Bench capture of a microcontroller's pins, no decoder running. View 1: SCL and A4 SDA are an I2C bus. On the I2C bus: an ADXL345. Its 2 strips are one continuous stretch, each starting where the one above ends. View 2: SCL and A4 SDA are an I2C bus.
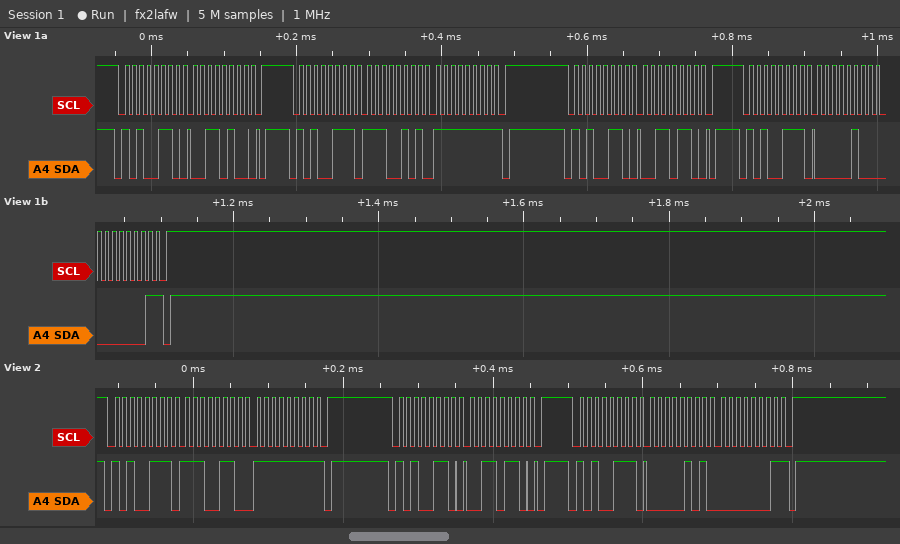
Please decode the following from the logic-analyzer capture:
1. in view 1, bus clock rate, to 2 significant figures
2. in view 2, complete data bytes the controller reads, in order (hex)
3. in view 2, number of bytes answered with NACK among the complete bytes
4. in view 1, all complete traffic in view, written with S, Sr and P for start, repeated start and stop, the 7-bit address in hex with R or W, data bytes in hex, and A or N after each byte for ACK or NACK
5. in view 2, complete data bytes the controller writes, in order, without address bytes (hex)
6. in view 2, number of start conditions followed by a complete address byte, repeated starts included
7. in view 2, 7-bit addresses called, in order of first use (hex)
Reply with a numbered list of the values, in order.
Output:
1. 100 kHz
2. E6 FF 05 01
3. 2
4. S 53W A 34 A P S 53R A E5 A FF N P S 53W A 36 A P S 53R A 04 A 01 N P
5. 36
6. 3
7. 0x53
